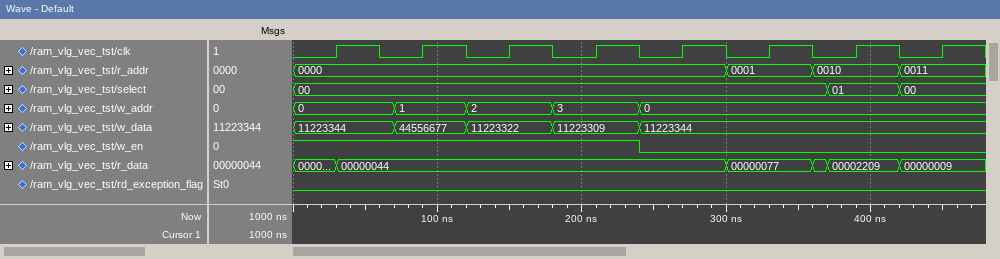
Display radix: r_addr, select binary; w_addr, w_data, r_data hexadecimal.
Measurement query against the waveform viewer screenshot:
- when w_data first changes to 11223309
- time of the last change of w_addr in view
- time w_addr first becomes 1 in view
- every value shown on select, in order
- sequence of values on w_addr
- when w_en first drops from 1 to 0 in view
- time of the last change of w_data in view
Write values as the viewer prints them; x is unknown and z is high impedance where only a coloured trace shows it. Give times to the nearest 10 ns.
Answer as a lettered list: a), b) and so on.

a) 180 ns
b) 240 ns
c) 70 ns
d) 00, 01, 00
e) 0, 1, 2, 3, 0
f) 240 ns
g) 240 ns
